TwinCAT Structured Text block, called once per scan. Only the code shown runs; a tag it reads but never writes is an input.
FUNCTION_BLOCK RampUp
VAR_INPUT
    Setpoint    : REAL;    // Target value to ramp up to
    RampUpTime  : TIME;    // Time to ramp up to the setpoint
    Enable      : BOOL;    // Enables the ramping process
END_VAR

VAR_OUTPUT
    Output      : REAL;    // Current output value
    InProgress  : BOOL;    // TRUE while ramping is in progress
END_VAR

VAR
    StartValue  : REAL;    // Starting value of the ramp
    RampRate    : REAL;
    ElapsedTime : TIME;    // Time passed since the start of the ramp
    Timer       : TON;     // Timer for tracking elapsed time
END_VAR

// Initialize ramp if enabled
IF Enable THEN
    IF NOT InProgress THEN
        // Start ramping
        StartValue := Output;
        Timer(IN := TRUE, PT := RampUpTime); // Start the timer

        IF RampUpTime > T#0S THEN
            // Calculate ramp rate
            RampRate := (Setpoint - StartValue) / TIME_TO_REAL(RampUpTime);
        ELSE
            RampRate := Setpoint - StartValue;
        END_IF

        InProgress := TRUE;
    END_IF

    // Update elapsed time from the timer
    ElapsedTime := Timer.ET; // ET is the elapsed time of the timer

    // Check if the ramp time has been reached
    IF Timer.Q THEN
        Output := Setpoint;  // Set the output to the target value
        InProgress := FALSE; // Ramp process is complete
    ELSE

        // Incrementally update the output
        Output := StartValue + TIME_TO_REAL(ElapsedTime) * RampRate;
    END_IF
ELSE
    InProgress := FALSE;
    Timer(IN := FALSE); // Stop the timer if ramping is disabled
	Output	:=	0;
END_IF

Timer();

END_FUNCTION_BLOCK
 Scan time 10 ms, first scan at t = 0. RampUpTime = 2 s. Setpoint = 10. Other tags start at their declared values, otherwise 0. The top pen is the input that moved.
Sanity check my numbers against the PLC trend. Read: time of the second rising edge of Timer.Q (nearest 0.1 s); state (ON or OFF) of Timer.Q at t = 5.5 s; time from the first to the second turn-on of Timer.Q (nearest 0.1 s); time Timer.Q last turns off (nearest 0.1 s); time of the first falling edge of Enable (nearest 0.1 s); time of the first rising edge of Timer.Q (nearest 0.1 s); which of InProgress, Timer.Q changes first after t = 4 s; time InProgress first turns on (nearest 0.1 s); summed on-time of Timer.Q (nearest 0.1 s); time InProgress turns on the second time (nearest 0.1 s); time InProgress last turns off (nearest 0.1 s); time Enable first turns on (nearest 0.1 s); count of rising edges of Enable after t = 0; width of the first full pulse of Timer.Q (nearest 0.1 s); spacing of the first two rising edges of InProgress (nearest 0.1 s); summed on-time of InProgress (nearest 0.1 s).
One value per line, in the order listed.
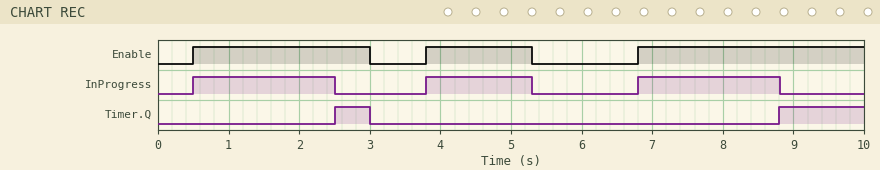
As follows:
8.8 s
OFF
6.3 s
3.0 s
3.0 s
2.5 s
InProgress
0.5 s
1.7 s
3.8 s
8.8 s
0.5 s
3
0.5 s
3.3 s
5.5 s
